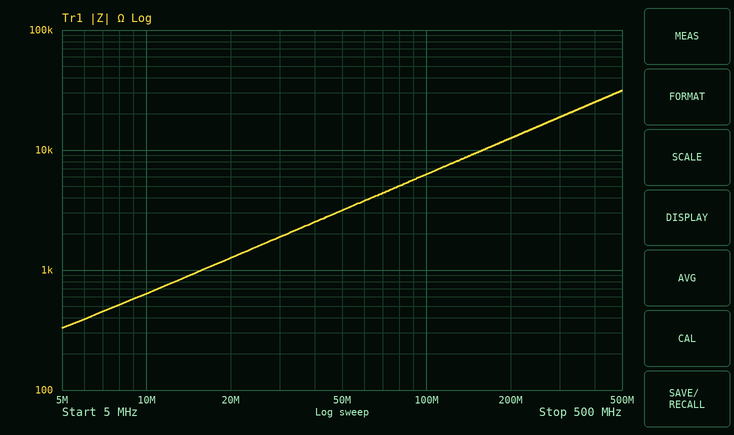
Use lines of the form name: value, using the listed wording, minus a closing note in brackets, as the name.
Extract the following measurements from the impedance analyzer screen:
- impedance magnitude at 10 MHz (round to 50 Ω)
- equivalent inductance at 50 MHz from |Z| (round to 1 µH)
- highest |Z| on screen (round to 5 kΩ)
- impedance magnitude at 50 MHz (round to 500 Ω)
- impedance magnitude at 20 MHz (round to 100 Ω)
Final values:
impedance magnitude at 10 MHz: 650 Ω
equivalent inductance at 50 MHz from |Z|: 10 µH
highest |Z| on screen: 30 kΩ
impedance magnitude at 50 MHz: 3.0 kΩ
impedance magnitude at 20 MHz: 1.3 kΩ
